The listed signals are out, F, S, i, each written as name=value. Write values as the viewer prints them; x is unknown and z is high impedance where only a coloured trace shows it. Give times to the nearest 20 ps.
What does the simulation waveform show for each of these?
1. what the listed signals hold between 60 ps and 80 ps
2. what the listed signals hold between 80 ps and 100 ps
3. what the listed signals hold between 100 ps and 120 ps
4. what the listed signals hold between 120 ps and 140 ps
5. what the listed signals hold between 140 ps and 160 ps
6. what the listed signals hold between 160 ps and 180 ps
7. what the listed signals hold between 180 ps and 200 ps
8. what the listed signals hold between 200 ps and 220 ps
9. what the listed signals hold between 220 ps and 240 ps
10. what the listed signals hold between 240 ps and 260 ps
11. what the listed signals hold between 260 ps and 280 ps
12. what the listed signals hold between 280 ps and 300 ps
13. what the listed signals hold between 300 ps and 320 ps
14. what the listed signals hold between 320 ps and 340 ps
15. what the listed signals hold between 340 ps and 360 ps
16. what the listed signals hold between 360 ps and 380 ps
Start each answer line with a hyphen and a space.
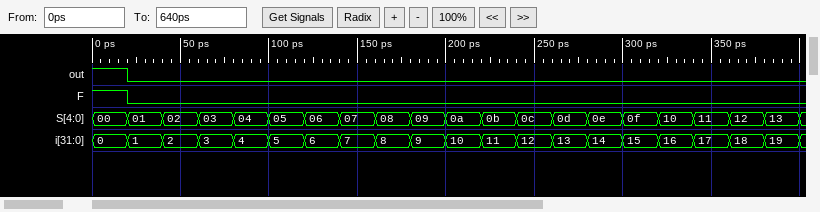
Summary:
- out=0, F=0, S=03, i=3
- out=0, F=0, S=04, i=4
- out=0, F=0, S=05, i=5
- out=0, F=0, S=06, i=6
- out=0, F=0, S=07, i=7
- out=0, F=0, S=08, i=8
- out=0, F=0, S=09, i=9
- out=0, F=0, S=0a, i=10
- out=0, F=0, S=0b, i=11
- out=0, F=0, S=0c, i=12
- out=0, F=0, S=0d, i=13
- out=0, F=0, S=0e, i=14
- out=0, F=0, S=0f, i=15
- out=0, F=0, S=10, i=16
- out=0, F=0, S=11, i=17
- out=0, F=0, S=12, i=18
